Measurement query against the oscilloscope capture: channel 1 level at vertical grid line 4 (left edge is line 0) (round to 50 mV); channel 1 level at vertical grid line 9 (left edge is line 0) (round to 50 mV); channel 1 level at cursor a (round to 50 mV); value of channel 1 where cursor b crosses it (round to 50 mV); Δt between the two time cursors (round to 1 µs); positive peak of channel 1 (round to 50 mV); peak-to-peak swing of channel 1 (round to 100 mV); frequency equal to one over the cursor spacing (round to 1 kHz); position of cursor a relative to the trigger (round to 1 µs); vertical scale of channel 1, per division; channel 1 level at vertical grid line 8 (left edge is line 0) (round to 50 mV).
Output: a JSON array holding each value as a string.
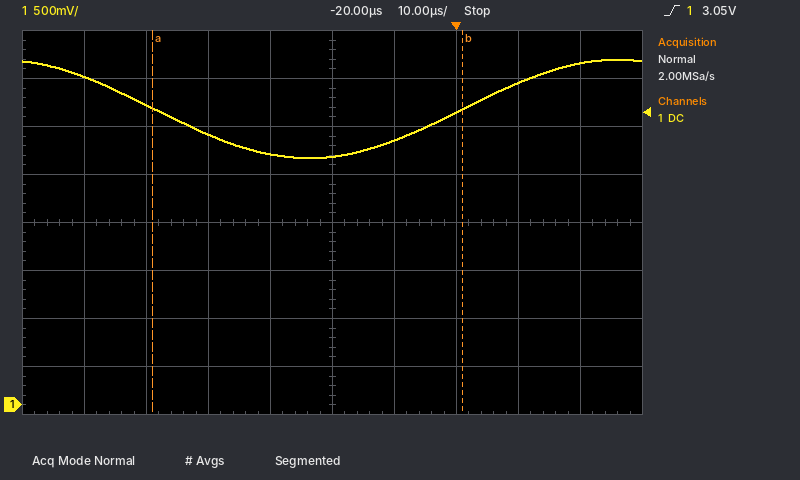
["2.60 V", "3.55 V", "3.10 V", "3.10 V", "50 µs", "3.60 V", "1.00 V", "20 kHz", "-49 µs", "500 mV", "3.35 V"]
